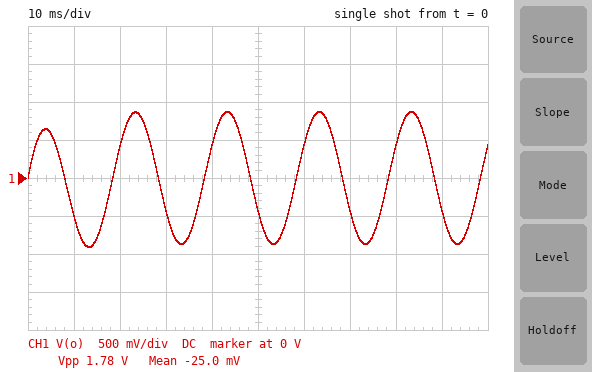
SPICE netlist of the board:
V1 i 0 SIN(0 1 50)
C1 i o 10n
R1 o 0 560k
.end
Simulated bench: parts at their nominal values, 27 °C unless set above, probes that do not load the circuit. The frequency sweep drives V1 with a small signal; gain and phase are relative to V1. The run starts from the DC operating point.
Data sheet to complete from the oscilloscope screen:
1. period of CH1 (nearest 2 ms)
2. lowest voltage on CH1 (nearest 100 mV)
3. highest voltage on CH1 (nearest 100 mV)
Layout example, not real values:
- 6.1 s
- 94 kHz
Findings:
- 20 ms
- -900 mV
- 900 mV
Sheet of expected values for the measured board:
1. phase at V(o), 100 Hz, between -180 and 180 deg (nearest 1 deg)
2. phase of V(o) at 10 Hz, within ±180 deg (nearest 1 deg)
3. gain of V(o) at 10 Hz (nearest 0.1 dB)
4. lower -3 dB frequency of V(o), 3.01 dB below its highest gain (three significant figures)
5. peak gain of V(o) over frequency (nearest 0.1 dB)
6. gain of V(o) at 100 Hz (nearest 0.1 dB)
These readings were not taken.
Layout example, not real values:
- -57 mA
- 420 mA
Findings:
- 16 deg
- 71 deg
- -9.6 dB
- 28.4 Hz
- 0 dB
- -0.3 dB
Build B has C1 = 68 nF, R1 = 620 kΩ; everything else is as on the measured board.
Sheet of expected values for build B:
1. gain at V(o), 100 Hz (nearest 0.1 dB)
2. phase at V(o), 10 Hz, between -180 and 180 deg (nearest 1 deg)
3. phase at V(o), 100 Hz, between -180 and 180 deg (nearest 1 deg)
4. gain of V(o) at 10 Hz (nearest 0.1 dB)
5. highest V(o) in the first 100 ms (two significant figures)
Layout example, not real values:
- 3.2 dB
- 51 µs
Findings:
- 0 dB
- 21 deg
- 2 deg
- -0.6 dB
- 990 mV
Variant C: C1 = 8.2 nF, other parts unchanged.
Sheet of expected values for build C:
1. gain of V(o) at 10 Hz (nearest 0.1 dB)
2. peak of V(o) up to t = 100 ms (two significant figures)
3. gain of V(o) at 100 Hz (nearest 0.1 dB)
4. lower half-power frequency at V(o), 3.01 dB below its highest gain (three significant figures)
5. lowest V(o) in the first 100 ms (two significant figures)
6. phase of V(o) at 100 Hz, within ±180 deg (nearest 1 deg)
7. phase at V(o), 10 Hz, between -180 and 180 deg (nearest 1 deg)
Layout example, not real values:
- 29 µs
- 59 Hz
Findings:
- -11.1 dB
- 820 mV
- -0.5 dB
- 34.7 Hz
- -850 mV
- 19 deg
- 74 deg
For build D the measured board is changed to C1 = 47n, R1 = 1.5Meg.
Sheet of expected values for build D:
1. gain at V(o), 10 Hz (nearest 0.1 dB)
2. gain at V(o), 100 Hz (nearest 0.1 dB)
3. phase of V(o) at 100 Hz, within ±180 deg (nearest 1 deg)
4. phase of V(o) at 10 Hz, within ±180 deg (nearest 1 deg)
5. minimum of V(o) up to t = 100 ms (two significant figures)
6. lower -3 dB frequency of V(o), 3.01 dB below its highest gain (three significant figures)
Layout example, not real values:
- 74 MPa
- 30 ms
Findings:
- -0.2 dB
- 0 dB
- 1 deg
- 13 deg
- -1.0 V
- 2.26 Hz
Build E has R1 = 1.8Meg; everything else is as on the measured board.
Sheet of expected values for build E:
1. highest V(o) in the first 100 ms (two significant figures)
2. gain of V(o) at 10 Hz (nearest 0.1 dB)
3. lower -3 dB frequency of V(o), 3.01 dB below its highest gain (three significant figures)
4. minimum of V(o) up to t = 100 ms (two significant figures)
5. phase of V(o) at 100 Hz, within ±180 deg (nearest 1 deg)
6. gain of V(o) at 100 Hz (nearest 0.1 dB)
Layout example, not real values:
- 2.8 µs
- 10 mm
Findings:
- 980 mV
- -2.5 dB
- 8.84 Hz
- -1.1 V
- 5 deg
- 0 dB
